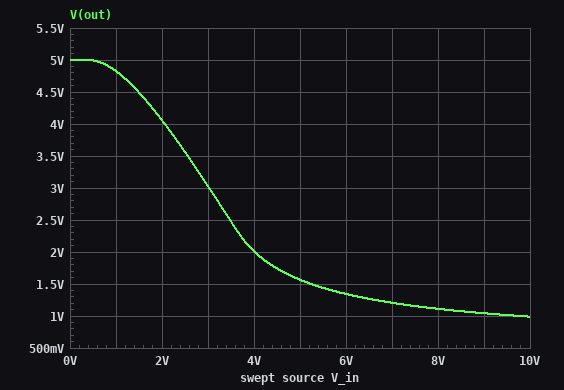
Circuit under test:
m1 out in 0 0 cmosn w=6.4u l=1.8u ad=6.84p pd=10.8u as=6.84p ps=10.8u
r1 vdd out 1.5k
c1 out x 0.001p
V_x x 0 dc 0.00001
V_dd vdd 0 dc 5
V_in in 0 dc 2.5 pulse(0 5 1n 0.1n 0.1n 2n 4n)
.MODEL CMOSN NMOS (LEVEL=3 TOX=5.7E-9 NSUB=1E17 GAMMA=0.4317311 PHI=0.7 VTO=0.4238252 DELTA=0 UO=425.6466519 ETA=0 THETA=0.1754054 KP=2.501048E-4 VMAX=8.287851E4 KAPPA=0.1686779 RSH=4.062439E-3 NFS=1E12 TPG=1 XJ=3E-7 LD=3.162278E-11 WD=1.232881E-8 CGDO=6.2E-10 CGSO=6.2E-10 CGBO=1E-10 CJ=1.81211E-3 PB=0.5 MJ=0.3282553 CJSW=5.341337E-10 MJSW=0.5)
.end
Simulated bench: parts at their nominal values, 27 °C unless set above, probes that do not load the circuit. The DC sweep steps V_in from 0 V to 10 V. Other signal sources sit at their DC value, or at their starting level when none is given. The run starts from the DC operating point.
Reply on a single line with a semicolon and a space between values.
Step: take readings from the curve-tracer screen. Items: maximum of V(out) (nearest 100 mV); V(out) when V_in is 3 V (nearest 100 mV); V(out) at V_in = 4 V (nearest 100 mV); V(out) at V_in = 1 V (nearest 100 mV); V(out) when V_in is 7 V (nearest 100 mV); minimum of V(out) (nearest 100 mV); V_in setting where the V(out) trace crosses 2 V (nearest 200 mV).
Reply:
5.0 V; 3.0 V; 2.0 V; 4.8 V; 1.2 V; 1.0 V; 4.0 V
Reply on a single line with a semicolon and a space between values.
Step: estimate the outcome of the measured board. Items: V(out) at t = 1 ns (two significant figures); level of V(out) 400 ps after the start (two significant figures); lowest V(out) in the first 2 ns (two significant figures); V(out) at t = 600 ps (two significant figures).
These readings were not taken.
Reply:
5.0 V; 5.0 V; 1.6 V; 5.0 V
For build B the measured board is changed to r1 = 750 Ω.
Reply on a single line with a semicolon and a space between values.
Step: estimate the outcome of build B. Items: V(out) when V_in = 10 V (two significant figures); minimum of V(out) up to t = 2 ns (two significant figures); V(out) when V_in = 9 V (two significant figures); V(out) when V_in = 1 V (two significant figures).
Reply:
1.8 V; 2.8 V; 1.9 V; 4.9 V
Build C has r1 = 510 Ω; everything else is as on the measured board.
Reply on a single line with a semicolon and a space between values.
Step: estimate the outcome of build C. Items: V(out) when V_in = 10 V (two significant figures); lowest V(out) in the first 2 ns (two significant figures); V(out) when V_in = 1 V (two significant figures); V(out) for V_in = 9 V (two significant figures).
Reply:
2.4 V; 3.5 V; 4.9 V; 2.5 V
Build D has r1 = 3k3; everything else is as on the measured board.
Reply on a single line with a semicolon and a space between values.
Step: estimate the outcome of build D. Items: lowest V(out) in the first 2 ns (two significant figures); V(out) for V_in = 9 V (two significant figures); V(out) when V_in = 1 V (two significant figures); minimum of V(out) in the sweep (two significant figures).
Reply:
700 mV; 490 mV; 4.6 V; 470 mV
